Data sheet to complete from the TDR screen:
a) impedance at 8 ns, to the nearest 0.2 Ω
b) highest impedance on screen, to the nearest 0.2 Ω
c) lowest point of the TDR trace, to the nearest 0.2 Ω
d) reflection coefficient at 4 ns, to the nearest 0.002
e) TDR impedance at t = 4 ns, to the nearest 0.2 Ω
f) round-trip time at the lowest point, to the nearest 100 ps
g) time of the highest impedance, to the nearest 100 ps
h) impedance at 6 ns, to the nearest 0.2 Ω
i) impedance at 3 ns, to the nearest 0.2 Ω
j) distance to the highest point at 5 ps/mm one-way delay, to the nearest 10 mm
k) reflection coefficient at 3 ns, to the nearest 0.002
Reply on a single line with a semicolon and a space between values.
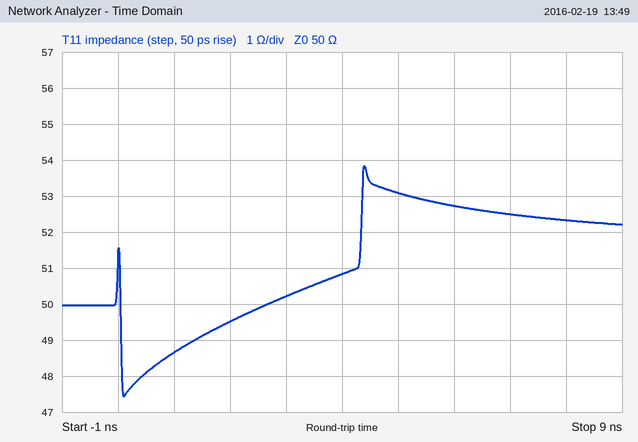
52.4 Ω; 53.8 Ω; 47.4 Ω; +0.008; 50.8 Ω; 100 ps; 4.4 ns; 52.8 Ω; 50.2 Ω; 440 mm; +0.002
